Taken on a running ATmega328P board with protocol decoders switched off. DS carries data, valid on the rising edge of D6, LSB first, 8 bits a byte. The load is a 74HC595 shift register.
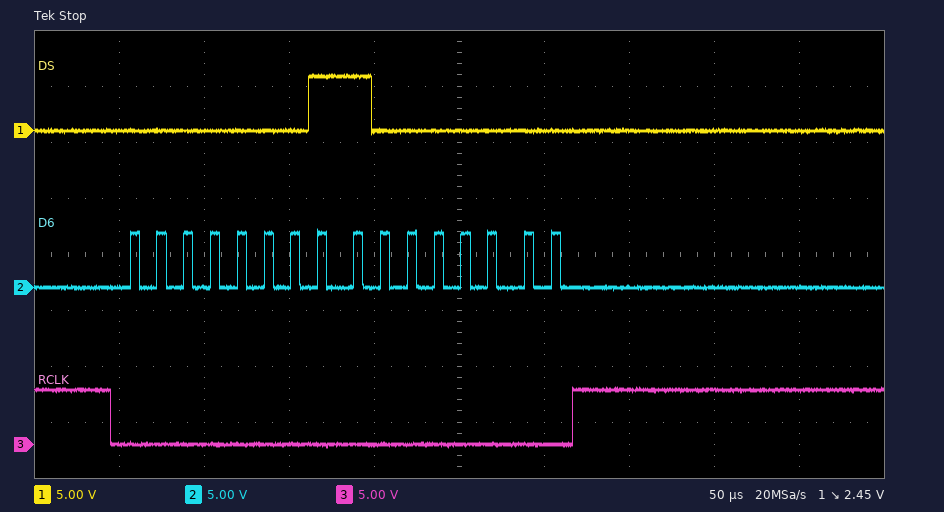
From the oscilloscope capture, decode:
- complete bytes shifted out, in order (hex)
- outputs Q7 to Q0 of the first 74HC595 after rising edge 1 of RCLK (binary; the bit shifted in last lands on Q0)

80 01
10000000
